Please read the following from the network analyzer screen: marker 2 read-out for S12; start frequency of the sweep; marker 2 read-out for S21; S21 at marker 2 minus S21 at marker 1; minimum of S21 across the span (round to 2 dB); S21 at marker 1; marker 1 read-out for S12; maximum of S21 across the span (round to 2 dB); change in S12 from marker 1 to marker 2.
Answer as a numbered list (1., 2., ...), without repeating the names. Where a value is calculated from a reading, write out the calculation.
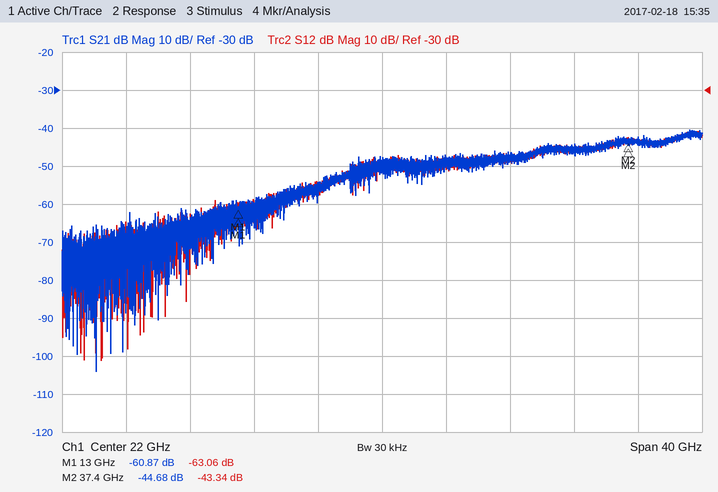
1. -43.34 dB
2. 2 GHz
3. -44.68 dB
4. -44.68 − (-60.87) = 16.19 dB
5. -104 dB
6. -60.87 dB
7. -63.06 dB
8. -40 dB
9. -43.34 − (-63.06) = 19.72 dB
